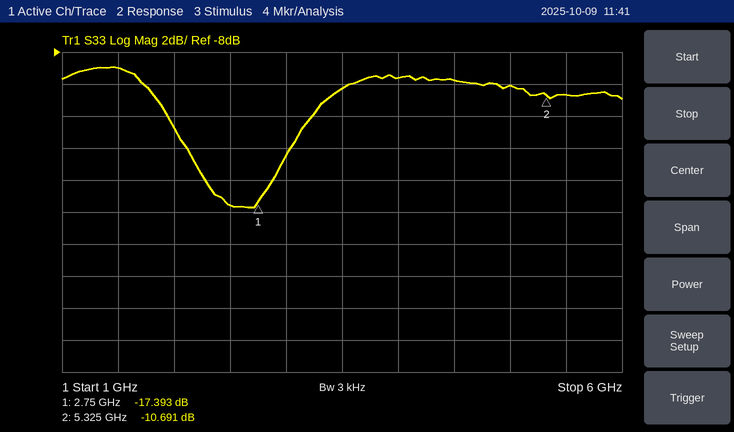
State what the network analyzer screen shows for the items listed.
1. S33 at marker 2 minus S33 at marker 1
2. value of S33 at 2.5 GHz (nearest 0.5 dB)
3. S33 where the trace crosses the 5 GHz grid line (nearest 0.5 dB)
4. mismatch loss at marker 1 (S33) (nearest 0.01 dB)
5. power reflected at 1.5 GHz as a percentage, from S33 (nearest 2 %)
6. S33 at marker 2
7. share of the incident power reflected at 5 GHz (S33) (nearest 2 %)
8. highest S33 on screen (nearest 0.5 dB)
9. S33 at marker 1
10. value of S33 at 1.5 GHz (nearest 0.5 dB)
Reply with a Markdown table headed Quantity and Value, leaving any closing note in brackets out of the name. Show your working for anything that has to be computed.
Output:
| Quantity | Value |
|---|---|
| S33 at marker 2 minus S33 at marker 1 | -10.691 − (-17.393) = 6.702 dB |
| value of S33 at 2.5 GHz | -17.5 dB |
| S33 where the trace crosses the 5 GHz grid line | -10.0 dB |
| mismatch loss at marker 1 (S33) | −10 log10(1 − 10^(-17.393/10)) ≈ 0.08 dB |
| power reflected at 1.5 GHz as a percentage, from S33 | 10^(-9/10) ≈ 12.6 %, so 12 % to the nearest 2 % |
| S33 at marker 2 | -10.691 dB |
| share of the incident power reflected at 5 GHz (S33) | 10^(-10/10) ≈ 10 % |
| highest S33 on screen | -9.0 dB |
| S33 at marker 1 | -17.393 dB |
| value of S33 at 1.5 GHz | -9.0 dB |
